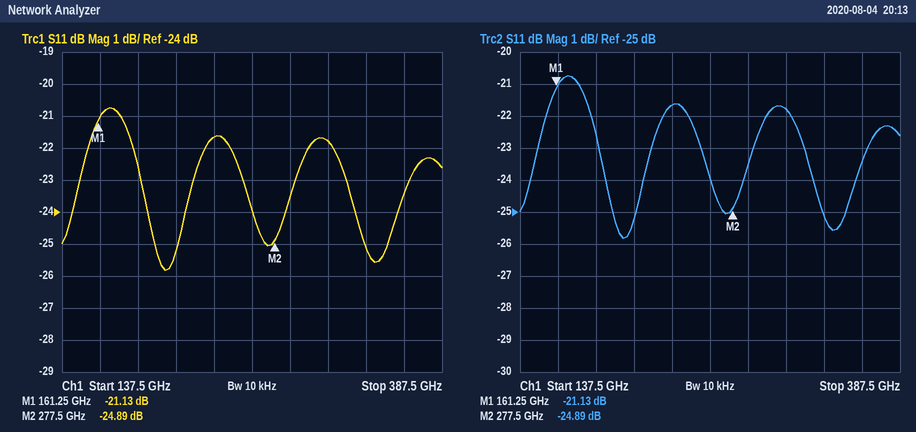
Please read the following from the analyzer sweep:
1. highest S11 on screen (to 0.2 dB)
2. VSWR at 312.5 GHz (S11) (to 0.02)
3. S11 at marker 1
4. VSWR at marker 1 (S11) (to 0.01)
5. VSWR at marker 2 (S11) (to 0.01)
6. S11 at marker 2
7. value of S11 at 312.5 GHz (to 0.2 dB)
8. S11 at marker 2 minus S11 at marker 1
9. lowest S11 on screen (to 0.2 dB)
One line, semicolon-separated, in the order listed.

-20.8 dB; 1.18; -21.13 dB; 1.19; 1.12; -24.89 dB; -21.8 dB; -3.76 dB; -25.8 dB
